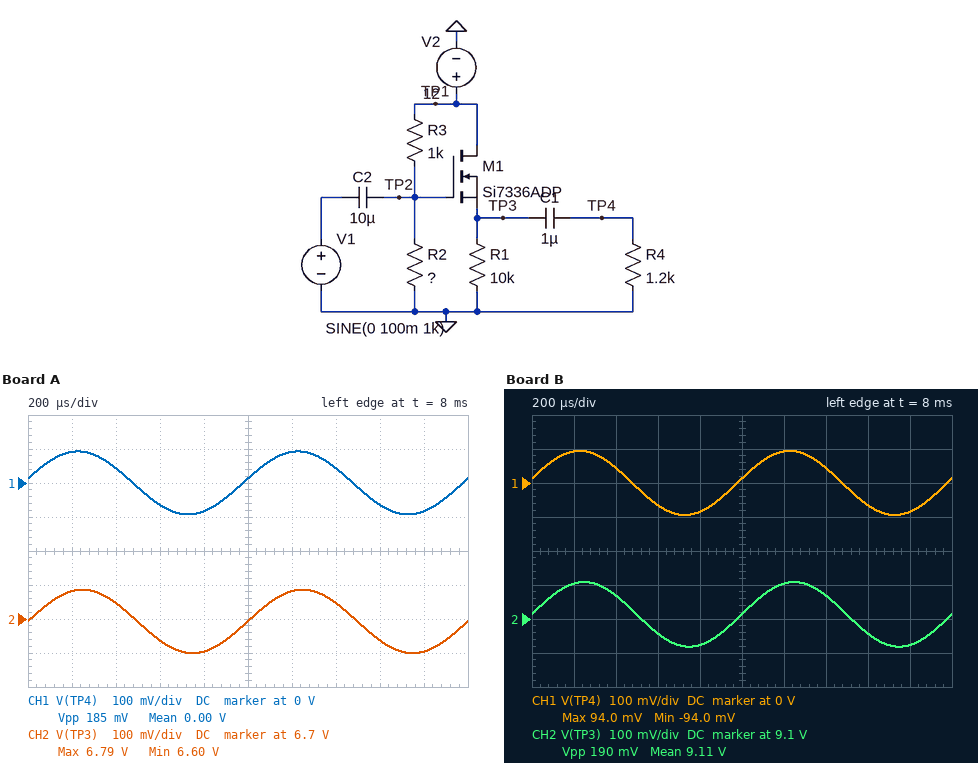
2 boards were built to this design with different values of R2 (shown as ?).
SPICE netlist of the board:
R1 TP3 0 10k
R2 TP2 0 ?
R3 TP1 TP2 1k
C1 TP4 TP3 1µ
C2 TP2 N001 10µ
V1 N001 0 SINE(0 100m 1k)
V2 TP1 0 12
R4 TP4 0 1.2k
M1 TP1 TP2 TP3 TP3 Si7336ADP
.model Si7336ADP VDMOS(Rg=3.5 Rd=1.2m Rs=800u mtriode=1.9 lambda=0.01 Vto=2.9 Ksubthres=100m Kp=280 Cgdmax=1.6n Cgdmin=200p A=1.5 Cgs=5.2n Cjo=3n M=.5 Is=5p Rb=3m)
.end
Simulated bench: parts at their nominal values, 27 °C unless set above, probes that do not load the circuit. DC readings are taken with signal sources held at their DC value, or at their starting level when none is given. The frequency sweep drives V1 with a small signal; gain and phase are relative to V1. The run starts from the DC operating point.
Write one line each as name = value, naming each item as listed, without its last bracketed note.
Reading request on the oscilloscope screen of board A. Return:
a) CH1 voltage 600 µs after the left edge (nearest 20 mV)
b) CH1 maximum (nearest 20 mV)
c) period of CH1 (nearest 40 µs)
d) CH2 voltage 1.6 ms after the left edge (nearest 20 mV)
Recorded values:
CH1 voltage 600 µs after the left edge = -60 mV
CH1 maximum = 100 mV
period of CH1 = 1.00 ms
CH2 voltage 1.6 ms after the left edge = 6.64 V
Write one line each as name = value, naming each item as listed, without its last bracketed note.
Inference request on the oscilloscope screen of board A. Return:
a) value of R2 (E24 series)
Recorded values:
value of R2 = 3.3 kΩ
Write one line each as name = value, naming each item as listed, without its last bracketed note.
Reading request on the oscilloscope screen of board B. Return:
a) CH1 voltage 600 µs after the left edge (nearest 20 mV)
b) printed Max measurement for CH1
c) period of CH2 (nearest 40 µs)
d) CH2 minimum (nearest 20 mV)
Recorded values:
CH1 voltage 600 µs after the left edge = -60 mV
printed Max measurement for CH1 = 94.0 mV
period of CH2 = 1.00 ms
CH2 minimum = 9.02 V
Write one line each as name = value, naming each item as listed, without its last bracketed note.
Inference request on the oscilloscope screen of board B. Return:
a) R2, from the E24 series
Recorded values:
R2, from the E24 series = 33 kΩ
